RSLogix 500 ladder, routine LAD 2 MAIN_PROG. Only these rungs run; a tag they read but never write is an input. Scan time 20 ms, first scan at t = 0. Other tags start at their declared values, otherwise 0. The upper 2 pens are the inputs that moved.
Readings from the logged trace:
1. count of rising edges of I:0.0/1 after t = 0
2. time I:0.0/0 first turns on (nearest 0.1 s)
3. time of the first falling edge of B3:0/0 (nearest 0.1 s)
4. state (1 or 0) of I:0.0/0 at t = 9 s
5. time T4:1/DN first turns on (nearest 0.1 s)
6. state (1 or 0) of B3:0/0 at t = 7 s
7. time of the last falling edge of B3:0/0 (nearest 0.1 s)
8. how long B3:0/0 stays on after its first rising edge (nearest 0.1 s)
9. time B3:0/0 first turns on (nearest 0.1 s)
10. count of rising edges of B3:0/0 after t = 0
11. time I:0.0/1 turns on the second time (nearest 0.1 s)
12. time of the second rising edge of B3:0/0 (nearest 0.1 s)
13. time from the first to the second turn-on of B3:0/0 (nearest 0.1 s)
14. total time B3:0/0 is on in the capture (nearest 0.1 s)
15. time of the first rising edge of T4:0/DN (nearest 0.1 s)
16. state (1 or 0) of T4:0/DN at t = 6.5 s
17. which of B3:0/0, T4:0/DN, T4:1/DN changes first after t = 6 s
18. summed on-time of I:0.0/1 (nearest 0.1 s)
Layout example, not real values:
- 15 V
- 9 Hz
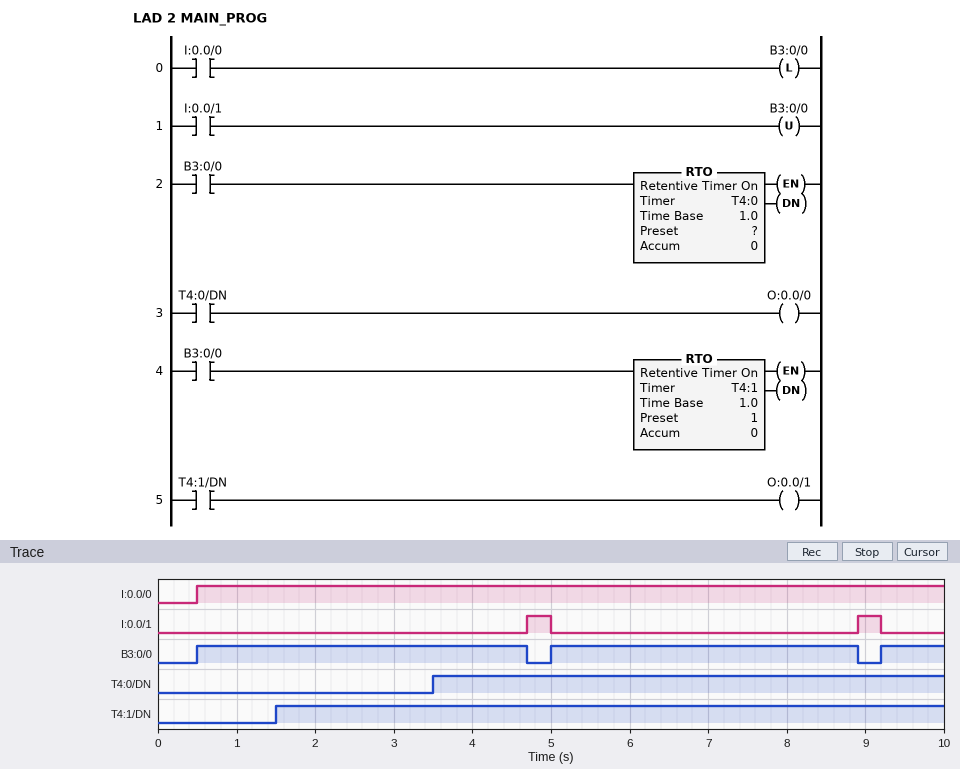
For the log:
- 2
- 0.5 s
- 4.7 s
- 1
- 1.5 s
- 1
- 8.9 s
- 4.2 s
- 0.5 s
- 3
- 8.9 s
- 5.0 s
- 4.5 s
- 8.9 s
- 3.5 s
- 1
- B3:0/0
- 0.6 s
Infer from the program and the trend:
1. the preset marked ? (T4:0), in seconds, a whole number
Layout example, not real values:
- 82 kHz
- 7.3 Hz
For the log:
- 3 s
